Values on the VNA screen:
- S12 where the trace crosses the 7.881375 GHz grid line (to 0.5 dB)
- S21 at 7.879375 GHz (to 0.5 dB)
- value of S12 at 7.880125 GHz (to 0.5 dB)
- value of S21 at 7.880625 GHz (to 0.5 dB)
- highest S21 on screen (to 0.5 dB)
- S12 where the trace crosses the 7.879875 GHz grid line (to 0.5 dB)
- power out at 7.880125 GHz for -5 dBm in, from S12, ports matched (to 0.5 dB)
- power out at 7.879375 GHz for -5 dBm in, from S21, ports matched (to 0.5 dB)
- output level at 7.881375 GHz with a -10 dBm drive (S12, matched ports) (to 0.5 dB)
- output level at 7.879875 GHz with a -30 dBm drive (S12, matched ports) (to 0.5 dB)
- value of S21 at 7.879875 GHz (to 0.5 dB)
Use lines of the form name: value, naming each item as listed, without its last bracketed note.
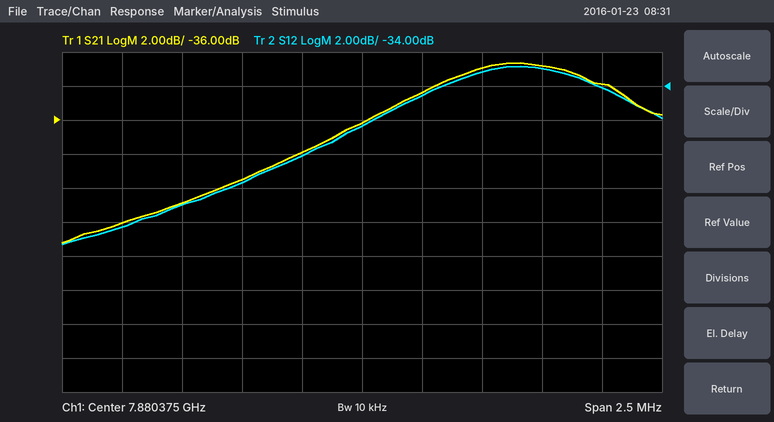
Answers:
S12 where the trace crosses the 7.881375 GHz grid line: -34.0 dB
S21 at 7.879375 GHz: -42.0 dB
value of S12 at 7.880125 GHz: -38.0 dB
value of S21 at 7.880625 GHz: -34.5 dB
highest S21 on screen: -32.5 dB
S12 where the trace crosses the 7.879875 GHz grid line: -39.5 dB
power out at 7.880125 GHz for -5 dBm in, from S12, ports matched: -43.0 dBm
power out at 7.879375 GHz for -5 dBm in, from S21, ports matched: -47.0 dBm
output level at 7.881375 GHz with a -10 dBm drive (S12, matched ports): -44.0 dBm
output level at 7.879875 GHz with a -30 dBm drive (S12, matched ports): -69.5 dBm
value of S21 at 7.879875 GHz: -39.5 dB
